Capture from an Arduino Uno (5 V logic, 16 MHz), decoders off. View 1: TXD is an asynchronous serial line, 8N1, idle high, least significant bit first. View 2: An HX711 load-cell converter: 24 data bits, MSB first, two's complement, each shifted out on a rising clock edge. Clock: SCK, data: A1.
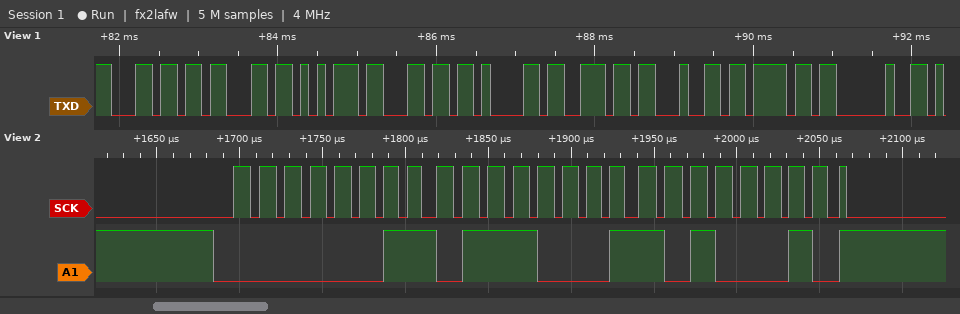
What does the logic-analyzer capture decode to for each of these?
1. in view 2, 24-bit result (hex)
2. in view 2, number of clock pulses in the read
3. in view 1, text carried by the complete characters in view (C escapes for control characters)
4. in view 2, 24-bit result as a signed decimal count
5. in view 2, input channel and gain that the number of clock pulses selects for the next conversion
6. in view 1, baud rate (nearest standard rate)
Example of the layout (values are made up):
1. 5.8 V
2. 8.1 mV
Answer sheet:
1. 0x0371A2
2. 25
3. "lculando "
4. 225698
5. channel A, gain 128
6. 9600 baud
